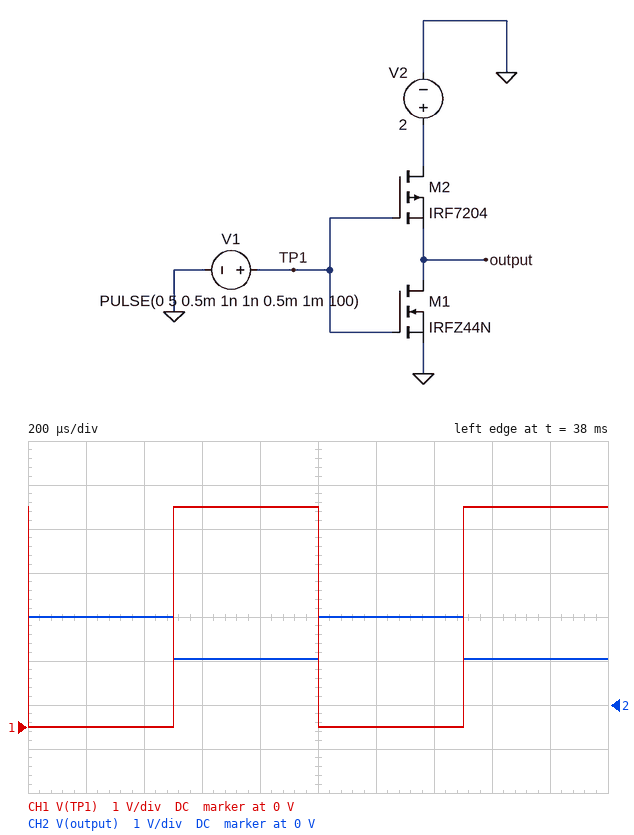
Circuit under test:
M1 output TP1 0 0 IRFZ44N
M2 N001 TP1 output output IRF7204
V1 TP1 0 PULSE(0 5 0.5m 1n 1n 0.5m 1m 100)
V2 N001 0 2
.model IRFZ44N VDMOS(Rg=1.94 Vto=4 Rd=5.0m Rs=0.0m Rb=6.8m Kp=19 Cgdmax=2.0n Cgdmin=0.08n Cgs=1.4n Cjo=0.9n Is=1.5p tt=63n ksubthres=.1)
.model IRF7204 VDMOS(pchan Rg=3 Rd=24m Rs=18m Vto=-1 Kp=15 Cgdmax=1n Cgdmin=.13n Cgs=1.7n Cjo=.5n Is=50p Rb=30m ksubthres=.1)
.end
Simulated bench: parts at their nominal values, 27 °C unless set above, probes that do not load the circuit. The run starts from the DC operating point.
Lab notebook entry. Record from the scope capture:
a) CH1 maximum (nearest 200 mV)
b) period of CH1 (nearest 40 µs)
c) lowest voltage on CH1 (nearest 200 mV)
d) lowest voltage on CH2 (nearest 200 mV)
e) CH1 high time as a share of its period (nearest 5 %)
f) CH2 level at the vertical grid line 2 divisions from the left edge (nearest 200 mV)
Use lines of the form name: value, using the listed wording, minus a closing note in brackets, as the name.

CH1 maximum: 5.0 V
period of CH1: 1.00 ms
lowest voltage on CH1: 0 V
lowest voltage on CH2: 1.0 V
CH1 high time as a share of its period: 50 %
CH2 level at the vertical grid line 2 divisions from the left edge: 2.0 V
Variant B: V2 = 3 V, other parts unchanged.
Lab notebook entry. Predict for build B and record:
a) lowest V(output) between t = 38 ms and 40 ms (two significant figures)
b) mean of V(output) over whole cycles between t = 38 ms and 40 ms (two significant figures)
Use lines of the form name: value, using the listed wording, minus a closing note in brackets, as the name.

lowest V(output) between t = 38 ms and 40 ms: 2.0 V
mean of V(output) over whole cycles between t = 38 ms and 40 ms: 2.5 V
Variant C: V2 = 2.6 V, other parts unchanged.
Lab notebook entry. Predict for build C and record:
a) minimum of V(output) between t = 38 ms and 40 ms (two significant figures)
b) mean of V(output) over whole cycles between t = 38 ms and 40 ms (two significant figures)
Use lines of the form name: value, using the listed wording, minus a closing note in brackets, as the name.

minimum of V(output) between t = 38 ms and 40 ms: 1.6 V
mean of V(output) over whole cycles between t = 38 ms and 40 ms: 2.1 V
